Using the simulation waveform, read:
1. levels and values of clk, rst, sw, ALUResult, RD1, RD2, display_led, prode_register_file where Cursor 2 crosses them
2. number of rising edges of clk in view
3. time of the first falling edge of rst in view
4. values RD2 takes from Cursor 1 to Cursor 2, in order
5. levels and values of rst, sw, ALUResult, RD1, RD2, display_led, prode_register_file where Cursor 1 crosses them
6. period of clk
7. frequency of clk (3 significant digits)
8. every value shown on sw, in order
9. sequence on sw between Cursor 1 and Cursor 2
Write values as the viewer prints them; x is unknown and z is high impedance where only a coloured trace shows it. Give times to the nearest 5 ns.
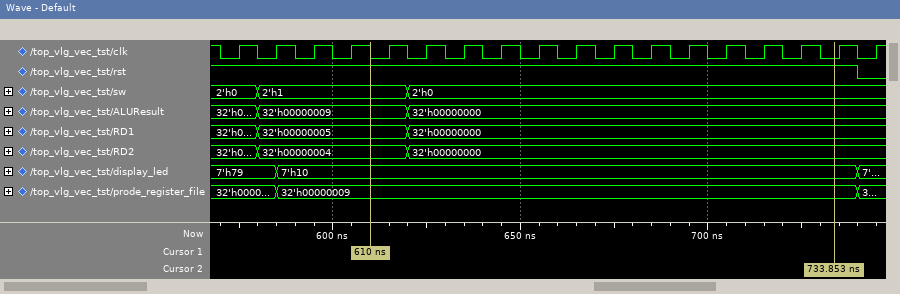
clk=0, rst=1, sw=2'h0, ALUResult=32'h00000000, RD1=32'h00000000, RD2=32'h00000000, display_led=7'h10, prode_register_file=32'h00000009
18
740 ns
32'h00000004, 32'h00000000
rst=1, sw=2'h1, ALUResult=32'h00000009, RD1=32'h00000005, RD2=32'h00000004, display_led=7'h10, prode_register_file=32'h00000009
10 ns
100 MHz
2'h0, 2'h1, 2'h0
2'h1, 2'h0
